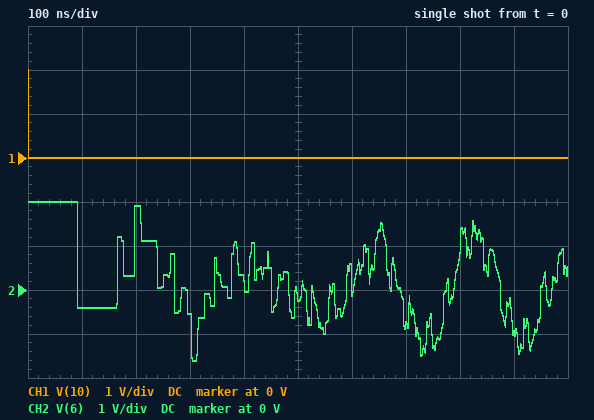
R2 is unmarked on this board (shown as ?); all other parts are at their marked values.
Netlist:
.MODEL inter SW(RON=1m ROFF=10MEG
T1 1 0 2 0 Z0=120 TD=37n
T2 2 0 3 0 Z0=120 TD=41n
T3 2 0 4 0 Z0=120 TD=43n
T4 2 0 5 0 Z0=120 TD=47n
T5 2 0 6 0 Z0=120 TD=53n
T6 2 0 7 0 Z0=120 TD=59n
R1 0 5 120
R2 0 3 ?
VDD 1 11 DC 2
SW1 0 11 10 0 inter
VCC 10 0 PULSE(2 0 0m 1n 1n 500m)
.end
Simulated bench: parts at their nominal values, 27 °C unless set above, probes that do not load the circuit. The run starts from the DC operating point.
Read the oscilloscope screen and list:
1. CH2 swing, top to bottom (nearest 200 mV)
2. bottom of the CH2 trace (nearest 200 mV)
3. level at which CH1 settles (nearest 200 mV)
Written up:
3.6 V
-1.6 V
0 V
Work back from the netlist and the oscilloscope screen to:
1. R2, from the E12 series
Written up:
150 Ω
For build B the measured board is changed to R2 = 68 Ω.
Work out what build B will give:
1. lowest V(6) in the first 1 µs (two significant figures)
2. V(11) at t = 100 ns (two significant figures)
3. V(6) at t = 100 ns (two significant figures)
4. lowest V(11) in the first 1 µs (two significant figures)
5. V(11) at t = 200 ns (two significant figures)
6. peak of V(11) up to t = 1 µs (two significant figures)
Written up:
-2.7 V
1.8 V
-1.7 V
-7.0 V
-6.4 V
3.1 V
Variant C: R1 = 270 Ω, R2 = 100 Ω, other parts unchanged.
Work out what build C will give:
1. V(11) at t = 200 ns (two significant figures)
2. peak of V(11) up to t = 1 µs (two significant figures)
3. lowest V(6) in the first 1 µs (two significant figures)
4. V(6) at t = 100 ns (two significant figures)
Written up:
-4.2 V
1.1 V
-1.5 V
-190 mV
